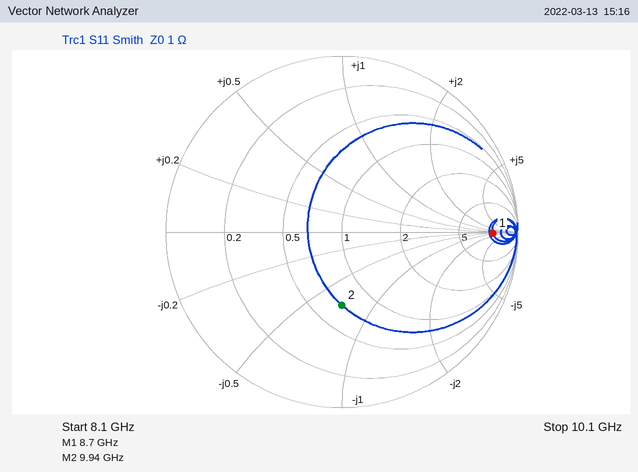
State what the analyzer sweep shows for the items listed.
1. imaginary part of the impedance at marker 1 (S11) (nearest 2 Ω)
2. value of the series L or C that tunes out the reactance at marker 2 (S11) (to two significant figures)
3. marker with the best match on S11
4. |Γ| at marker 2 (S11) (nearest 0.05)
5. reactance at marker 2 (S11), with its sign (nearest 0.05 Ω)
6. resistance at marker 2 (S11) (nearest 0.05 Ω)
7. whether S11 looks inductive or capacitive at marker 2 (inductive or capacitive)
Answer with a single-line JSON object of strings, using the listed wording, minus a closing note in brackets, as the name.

{"imaginary part of the impedance at marker 1 (S11)": "0 Ω", "value of the series L or C that tunes out the reactance at marker 2 (S11)": "11 pH", "marker with the best match on S11": "marker 2", "|Γ| at marker 2 (S11)": "0.40", "reactance at marker 2 (S11), with its sign": "-0.70 Ω", "resistance at marker 2 (S11)": "0.70 Ω", "whether S11 looks inductive or capacitive at marker 2": "capacitive"}
